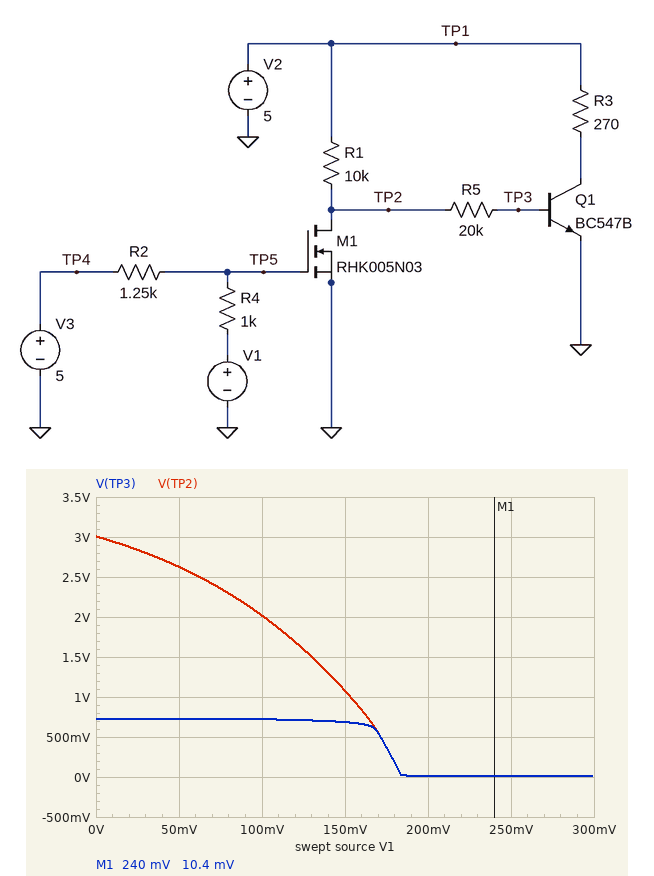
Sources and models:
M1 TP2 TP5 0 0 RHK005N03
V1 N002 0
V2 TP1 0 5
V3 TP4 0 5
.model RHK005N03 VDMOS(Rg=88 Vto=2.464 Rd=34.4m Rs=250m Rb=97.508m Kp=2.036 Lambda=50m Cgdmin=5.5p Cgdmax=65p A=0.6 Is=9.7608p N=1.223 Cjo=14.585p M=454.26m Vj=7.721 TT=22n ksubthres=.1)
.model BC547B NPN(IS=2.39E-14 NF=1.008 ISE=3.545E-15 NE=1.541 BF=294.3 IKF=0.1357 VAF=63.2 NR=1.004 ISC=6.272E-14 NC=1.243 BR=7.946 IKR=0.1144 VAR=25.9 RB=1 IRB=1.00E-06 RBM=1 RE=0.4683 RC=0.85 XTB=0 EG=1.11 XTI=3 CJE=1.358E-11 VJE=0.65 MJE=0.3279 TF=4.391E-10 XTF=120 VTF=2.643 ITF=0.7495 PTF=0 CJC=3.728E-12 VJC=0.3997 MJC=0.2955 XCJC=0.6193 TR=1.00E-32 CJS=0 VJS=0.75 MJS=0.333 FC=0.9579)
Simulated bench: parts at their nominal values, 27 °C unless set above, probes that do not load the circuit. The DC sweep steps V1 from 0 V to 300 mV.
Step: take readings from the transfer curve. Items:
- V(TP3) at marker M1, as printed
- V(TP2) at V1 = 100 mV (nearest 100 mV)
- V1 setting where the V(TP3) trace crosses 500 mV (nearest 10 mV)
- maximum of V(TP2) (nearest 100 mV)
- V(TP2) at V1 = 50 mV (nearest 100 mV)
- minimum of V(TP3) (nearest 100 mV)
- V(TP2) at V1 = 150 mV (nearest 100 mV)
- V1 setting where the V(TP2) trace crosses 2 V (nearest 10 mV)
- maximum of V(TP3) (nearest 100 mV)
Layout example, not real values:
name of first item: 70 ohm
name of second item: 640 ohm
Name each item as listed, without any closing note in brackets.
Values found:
V(TP3) at marker M1, as printed: 10.4 mV
V(TP2) at V1 = 100 mV: 2.0 V
V1 setting where the V(TP3) trace crosses 500 mV: 170 mV
maximum of V(TP2): 3.0 V
V(TP2) at V1 = 50 mV: 2.6 V
minimum of V(TP3): 0 V
V(TP2) at V1 = 150 mV: 1.1 V
V1 setting where the V(TP2) trace crosses 2 V: 100 mV
maximum of V(TP3): 700 mV
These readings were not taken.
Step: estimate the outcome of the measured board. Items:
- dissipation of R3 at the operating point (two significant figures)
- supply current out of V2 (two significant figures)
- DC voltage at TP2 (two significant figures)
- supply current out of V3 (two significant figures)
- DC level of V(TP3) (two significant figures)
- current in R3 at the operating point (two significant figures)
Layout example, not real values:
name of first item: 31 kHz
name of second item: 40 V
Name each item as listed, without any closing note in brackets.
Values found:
dissipation of R3 at the operating point: 87 mW
supply current out of V2: 18 mA
DC voltage at TP2: 3.0 V
supply current out of V3: 2.2 mA
DC level of V(TP3): 730 mV
current in R3 at the operating point: 18 mA
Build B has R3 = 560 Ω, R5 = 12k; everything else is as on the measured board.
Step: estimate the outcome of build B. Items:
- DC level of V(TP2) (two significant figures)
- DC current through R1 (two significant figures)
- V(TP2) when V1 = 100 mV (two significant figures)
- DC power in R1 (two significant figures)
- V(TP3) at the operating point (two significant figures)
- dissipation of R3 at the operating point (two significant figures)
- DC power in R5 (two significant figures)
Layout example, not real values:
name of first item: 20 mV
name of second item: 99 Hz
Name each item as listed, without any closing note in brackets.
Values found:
DC level of V(TP2): 2.6 V
DC current through R1: 240 µA
V(TP2) when V1 = 100 mV: 1.8 V
DC power in R1: 580 µW
V(TP3) at the operating point: 700 mV
dissipation of R3 at the operating point: 43 mW
DC power in R5: 300 µW
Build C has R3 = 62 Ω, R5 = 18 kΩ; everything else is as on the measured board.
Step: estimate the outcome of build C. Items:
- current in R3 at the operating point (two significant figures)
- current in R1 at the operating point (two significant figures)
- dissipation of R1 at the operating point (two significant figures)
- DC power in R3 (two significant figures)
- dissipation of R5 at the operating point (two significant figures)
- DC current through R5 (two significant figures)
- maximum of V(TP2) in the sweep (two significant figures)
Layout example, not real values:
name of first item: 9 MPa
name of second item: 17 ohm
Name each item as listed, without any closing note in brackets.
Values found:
current in R3 at the operating point: 30 mA
current in R1 at the operating point: 210 µA
dissipation of R1 at the operating point: 430 µW
DC power in R3: 54 mW
dissipation of R5 at the operating point: 270 µW
DC current through R5: 120 µA
maximum of V(TP2) in the sweep: 2.9 V
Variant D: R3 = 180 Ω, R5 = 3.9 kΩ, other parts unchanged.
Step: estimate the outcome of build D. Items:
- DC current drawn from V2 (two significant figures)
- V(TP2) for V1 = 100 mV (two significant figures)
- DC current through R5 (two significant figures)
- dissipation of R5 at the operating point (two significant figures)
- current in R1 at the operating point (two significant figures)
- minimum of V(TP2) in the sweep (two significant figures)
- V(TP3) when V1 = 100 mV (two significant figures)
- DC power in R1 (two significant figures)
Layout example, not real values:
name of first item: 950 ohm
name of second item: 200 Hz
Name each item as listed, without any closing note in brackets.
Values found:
DC current drawn from V2: 27 mA
V(TP2) for V1 = 100 mV: 1.3 V
DC current through R5: 250 µA
dissipation of R5 at the operating point: 240 µW
current in R1 at the operating point: 330 µA
minimum of V(TP2) in the sweep: 7.1 mV
V(TP3) when V1 = 100 mV: 740 mV
DC power in R1: 1.1 mW
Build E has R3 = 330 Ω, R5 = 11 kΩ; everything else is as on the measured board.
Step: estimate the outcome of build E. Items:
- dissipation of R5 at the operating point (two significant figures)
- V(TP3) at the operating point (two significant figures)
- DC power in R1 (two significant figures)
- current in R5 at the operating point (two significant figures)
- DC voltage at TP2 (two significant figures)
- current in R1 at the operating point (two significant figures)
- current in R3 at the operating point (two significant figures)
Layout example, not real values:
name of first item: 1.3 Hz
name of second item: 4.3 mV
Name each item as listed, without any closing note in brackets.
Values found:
dissipation of R5 at the operating point: 300 µW
V(TP3) at the operating point: 720 mV
DC power in R1: 610 µW
current in R5 at the operating point: 160 µA
DC voltage at TP2: 2.5 V
current in R1 at the operating point: 250 µA
current in R3 at the operating point: 15 mA
